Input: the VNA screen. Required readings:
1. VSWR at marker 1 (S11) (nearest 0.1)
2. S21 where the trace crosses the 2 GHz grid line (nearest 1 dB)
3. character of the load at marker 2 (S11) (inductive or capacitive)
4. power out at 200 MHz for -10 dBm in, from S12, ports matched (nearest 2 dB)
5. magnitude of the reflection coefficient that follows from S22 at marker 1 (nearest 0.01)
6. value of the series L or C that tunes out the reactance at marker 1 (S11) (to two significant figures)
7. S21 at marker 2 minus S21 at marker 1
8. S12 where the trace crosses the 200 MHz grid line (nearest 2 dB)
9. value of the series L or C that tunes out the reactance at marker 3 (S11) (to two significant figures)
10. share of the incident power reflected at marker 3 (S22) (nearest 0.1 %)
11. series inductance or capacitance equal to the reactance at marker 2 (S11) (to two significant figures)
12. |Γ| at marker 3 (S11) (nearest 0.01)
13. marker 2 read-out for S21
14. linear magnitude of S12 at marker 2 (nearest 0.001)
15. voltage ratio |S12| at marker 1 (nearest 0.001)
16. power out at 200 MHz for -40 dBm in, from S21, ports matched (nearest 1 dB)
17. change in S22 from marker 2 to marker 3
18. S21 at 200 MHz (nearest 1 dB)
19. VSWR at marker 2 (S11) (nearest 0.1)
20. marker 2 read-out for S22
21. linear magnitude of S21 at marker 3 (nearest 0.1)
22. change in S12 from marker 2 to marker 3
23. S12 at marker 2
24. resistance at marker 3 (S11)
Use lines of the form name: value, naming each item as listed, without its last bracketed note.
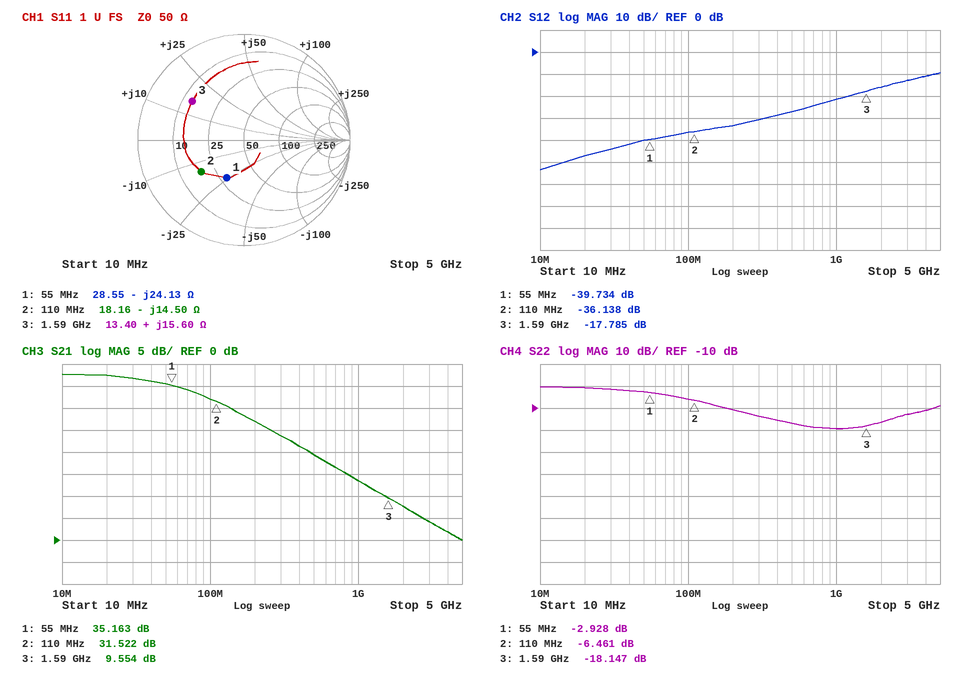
VSWR at marker 1 (S11): 2.3
S21 where the trace crosses the 2 GHz grid line: 8 dB
character of the load at marker 2 (S11): capacitive
power out at 200 MHz for -10 dBm in, from S12, ports matched: -44 dBm
magnitude of the reflection coefficient that follows from S22 at marker 1: 0.71
value of the series L or C that tunes out the reactance at marker 1 (S11): 70 nH
S21 at marker 2 minus S21 at marker 1: -3.641 dB
S12 where the trace crosses the 200 MHz grid line: -34 dB
value of the series L or C that tunes out the reactance at marker 3 (S11): 6.4 pF
share of the incident power reflected at marker 3 (S22): 1.5 %
series inductance or capacitance equal to the reactance at marker 2 (S11): 100 pF
|Γ| at marker 3 (S11): 0.61
marker 2 read-out for S21: 31.522 dB
linear magnitude of S12 at marker 2: 0.016
voltage ratio |S12| at marker 1: 0.010
power out at 200 MHz for -40 dBm in, from S21, ports matched: -13 dBm
change in S22 from marker 2 to marker 3: -11.686 dB
S21 at 200 MHz: 27 dB
VSWR at marker 2 (S11): 3.0
marker 2 read-out for S22: -6.461 dB
linear magnitude of S21 at marker 3: 3.0
change in S12 from marker 2 to marker 3: 18.353 dB
S12 at marker 2: -36.138 dB
resistance at marker 3: 13.40 Ω
